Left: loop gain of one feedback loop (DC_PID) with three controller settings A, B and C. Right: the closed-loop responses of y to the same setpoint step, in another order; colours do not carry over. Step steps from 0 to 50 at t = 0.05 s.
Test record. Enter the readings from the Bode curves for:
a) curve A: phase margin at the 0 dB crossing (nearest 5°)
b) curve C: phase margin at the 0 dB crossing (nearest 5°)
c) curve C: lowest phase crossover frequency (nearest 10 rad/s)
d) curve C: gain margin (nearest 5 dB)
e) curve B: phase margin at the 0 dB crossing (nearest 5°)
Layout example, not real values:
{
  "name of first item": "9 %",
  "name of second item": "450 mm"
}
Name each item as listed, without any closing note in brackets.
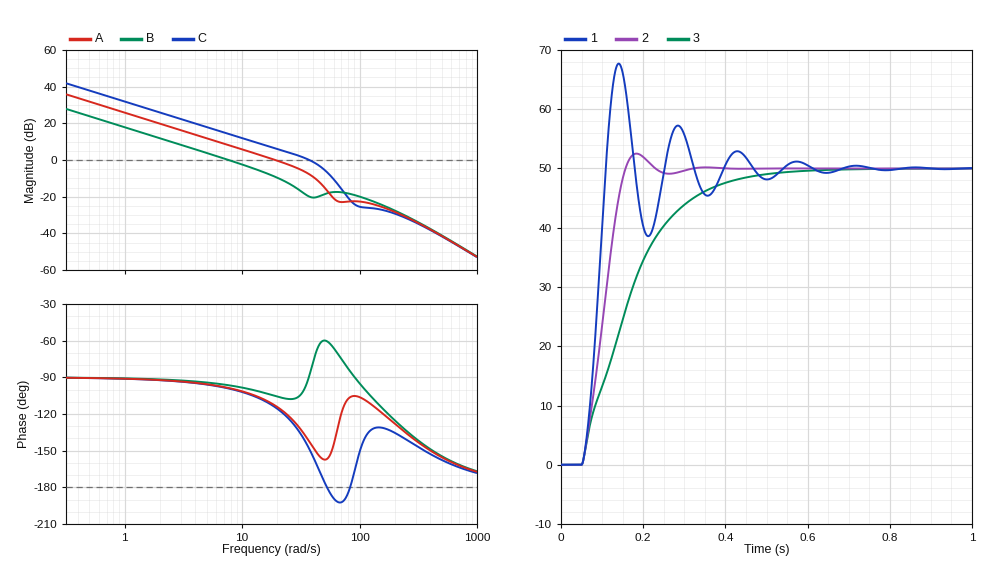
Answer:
{
  "curve A: phase margin at the 0 dB crossing": "65°",
  "curve C: phase margin at the 0 dB crossing": "30°",
  "curve C: lowest phase crossover frequency": "50 rad/s",
  "curve C: gain margin": "5 dB",
  "curve B: phase margin at the 0 dB crossing": "85°"
}
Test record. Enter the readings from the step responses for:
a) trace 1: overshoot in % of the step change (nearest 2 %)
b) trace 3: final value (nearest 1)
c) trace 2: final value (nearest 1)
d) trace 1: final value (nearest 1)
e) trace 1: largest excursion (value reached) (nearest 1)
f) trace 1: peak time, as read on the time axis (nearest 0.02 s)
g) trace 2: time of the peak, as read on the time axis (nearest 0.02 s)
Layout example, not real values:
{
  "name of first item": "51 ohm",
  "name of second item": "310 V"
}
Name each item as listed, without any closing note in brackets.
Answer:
{
  "trace 1: overshoot in % of the step change": "36 %",
  "trace 3: final value": "50",
  "trace 2: final value": "50",
  "trace 1: final value": "50",
  "trace 1: largest excursion (value reached)": "68",
  "trace 1: peak time, as read on the time axis": "0.14 s",
  "trace 2: time of the peak, as read on the time axis": "0.18 s"
}
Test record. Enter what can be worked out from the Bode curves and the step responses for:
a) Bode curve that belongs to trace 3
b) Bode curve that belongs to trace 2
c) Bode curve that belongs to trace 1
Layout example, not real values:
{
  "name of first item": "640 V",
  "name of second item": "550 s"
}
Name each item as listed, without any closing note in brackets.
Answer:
{
  "Bode curve that belongs to trace 3": "B",
  "Bode curve that belongs to trace 2": "A",
  "Bode curve that belongs to trace 1": "C"
}
